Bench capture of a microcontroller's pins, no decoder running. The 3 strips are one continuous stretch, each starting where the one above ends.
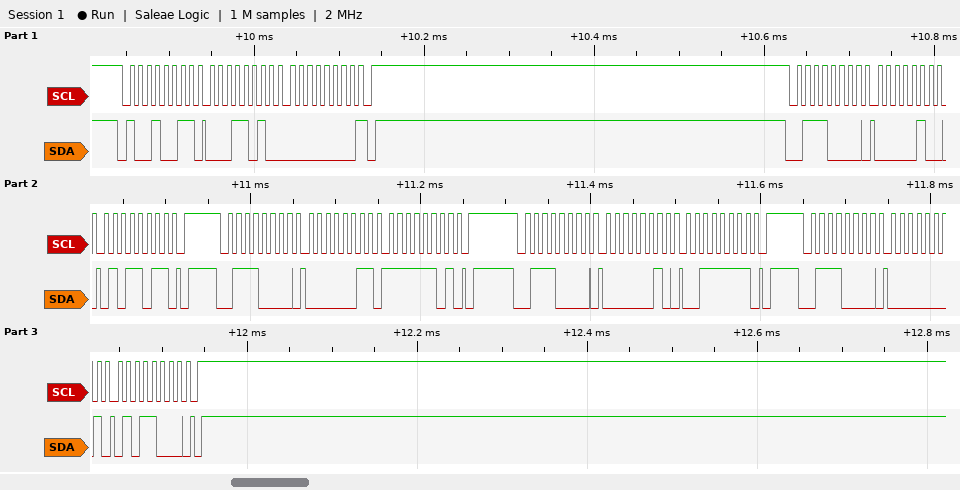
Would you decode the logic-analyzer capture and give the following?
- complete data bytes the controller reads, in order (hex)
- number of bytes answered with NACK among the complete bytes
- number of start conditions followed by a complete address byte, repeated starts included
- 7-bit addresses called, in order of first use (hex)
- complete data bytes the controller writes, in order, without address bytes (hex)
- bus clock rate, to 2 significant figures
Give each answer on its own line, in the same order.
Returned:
1A 00
1
5
0x49 0x38
04 5B 03 FD 02 3F 01 58
100 kHz
